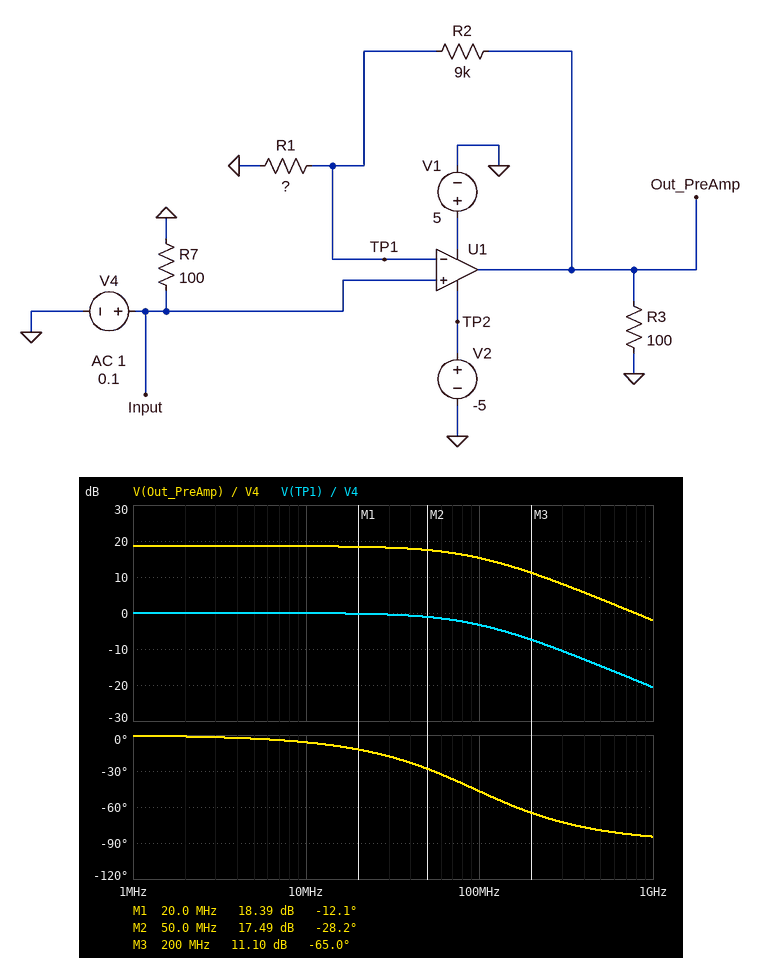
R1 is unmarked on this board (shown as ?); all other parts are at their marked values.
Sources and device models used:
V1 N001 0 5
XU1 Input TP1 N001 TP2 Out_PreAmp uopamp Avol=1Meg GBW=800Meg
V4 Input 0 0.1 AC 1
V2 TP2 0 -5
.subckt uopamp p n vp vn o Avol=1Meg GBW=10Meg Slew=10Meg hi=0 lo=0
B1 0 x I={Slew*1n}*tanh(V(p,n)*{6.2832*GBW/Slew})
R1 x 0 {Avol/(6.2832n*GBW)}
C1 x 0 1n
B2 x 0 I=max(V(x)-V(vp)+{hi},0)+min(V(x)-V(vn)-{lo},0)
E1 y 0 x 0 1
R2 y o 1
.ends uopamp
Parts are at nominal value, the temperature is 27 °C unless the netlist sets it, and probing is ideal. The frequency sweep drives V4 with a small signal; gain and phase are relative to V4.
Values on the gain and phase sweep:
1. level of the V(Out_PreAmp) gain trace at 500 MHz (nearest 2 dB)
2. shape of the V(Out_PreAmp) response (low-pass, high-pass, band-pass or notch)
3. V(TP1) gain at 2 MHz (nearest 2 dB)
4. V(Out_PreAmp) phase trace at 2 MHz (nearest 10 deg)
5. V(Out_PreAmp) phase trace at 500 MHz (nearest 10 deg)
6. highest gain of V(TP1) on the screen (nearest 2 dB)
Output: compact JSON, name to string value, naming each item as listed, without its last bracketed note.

{"level of the V(Out_PreAmp) gain trace at 500 MHz": "4 dB", "shape of the V(Out_PreAmp) response": "low-pass", "V(TP1) gain at 2 MHz": "0 dB", "V(Out_PreAmp) phase trace at 2 MHz": "0 deg", "V(Out_PreAmp) phase trace at 500 MHz": "-80 deg", "highest gain of V(TP1) on the screen": "0 dB"}
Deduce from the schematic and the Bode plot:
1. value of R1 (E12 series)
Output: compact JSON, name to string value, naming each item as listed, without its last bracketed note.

{"value of R1": "1.2 kΩ"}
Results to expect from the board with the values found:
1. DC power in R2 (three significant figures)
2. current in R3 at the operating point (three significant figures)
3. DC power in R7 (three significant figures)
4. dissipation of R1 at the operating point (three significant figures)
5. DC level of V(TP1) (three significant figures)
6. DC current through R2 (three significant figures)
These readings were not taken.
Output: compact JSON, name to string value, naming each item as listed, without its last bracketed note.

{"DC power in R2": "62.5 µW", "current in R3 at the operating point": "8.50 mA", "DC power in R7": "100 µW", "dissipation of R1 at the operating point": "8.33 µW", "DC level of V(TP1)": "100 mV", "DC current through R2": "83.3 µA"}
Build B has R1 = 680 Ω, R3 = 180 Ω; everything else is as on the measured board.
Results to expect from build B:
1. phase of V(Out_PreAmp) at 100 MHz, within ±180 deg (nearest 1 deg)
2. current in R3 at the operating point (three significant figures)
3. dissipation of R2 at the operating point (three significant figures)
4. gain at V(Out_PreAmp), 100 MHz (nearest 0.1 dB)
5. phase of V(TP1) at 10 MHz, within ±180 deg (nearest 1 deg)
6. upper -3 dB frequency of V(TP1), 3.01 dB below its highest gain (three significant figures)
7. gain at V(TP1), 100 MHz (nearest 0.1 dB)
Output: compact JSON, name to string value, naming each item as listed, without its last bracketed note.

{"phase of V(Out_PreAmp) at 100 MHz, within ±180 deg": "-61 deg", "current in R3 at the operating point": "7.91 mA", "dissipation of R2 at the operating point": "195 µW", "gain at V(Out_PreAmp), 100 MHz": "16.8 dB", "phase of V(TP1) at 10 MHz, within ±180 deg": "-10 deg", "upper -3 dB frequency of V(TP1), 3.01 dB below its highest gain": "55.9 MHz", "gain at V(TP1), 100 MHz": "-6.2 dB"}
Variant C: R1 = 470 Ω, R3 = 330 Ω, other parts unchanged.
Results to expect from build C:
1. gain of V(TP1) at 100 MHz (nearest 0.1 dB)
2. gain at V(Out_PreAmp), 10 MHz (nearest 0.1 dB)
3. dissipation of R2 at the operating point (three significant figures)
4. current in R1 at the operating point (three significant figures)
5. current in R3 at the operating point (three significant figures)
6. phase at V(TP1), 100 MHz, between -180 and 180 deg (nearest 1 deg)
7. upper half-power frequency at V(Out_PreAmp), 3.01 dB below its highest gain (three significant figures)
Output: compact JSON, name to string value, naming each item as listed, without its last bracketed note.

{"gain of V(TP1) at 100 MHz": "-8.7 dB", "gain at V(Out_PreAmp), 10 MHz": "25.8 dB", "dissipation of R2 at the operating point": "407 µW", "current in R1 at the operating point": "213 µA", "current in R3 at the operating point": "6.11 mA", "phase at V(TP1), 100 MHz, between -180 and 180 deg": "-68 deg", "upper half-power frequency at V(Out_PreAmp), 3.01 dB below its highest gain": "39.6 MHz"}
